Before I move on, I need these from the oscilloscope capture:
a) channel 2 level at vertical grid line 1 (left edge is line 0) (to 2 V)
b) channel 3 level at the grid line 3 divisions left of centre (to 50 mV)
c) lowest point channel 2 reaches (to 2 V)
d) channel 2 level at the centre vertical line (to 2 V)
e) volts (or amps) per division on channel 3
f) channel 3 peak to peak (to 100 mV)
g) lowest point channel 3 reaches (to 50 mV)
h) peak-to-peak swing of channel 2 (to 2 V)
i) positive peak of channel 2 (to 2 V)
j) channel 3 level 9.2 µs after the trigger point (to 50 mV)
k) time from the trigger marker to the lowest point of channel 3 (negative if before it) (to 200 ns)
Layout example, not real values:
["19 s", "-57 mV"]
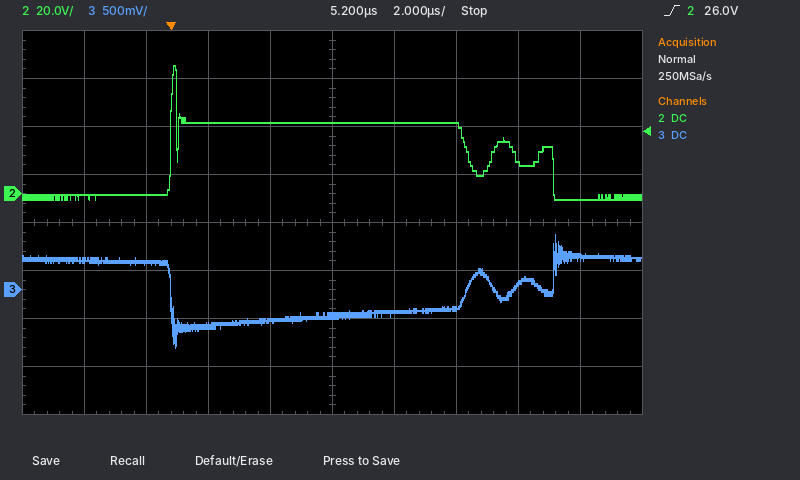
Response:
["0 V", "300 mV", "-2 V", "30 V", "500 mV", "1.20 V", "-600 mV", "56 V", "54 V", "-200 mV", "+200 ns"]
